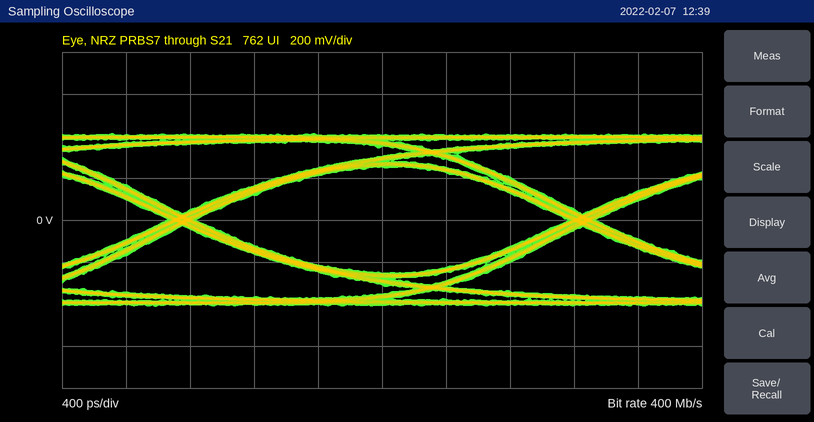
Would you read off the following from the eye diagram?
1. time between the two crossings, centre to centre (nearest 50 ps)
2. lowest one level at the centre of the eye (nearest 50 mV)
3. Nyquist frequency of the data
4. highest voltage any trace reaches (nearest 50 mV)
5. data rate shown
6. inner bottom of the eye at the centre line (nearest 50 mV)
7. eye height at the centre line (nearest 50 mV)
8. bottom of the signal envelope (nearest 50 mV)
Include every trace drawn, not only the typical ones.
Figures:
2.50 ns
250 mV
200 MHz
400 mV
400 Mb/s
-250 mV
500 mV
-400 mV
